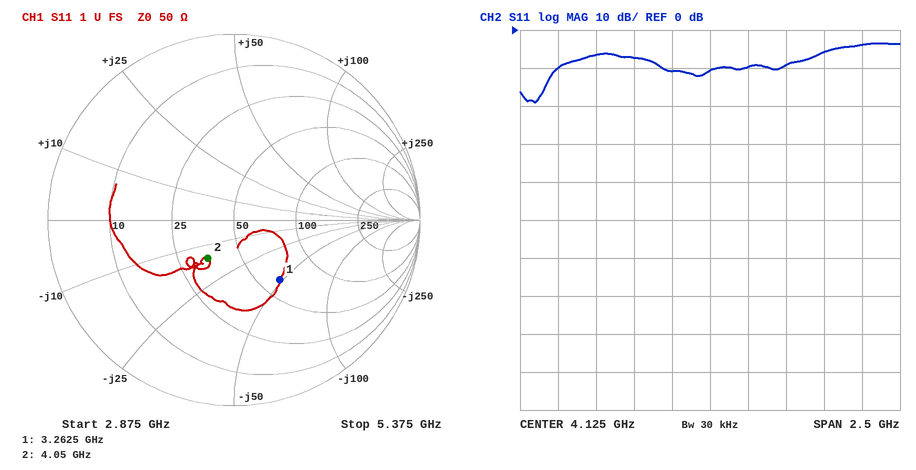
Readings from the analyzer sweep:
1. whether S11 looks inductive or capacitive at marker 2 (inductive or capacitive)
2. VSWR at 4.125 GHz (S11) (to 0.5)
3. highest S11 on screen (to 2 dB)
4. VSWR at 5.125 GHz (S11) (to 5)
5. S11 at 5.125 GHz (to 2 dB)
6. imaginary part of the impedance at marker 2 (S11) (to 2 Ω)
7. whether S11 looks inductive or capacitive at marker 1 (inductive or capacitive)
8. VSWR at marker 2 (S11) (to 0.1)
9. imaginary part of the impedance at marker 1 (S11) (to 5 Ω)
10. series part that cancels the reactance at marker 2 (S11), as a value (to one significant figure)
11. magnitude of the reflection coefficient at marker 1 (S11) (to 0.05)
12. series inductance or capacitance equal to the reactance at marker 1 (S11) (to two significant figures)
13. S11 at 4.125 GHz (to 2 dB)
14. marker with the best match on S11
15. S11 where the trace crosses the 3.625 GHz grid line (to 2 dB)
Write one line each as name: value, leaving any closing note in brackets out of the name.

whether S11 looks inductive or capacitive at marker 2: capacitive
VSWR at 4.125 GHz (S11): 2.0
highest S11 on screen: -4 dB
VSWR at 5.125 GHz (S11): 5
S11 at 5.125 GHz: -4 dB
imaginary part of the impedance at marker 2 (S11): -16 Ω
whether S11 looks inductive or capacitive at marker 1: capacitive
VSWR at marker 2 (S11): 1.7
imaginary part of the impedance at marker 1 (S11): -50 Ω
series part that cancels the reactance at marker 2 (S11), as a value: 600 pH
magnitude of the reflection coefficient at marker 1 (S11): 0.40
series inductance or capacitance equal to the reactance at marker 1 (S11): 1.0 pF
S11 at 4.125 GHz: -10 dB
marker with the best match on S11: marker 2
S11 where the trace crosses the 3.625 GHz grid line: -8 dB
